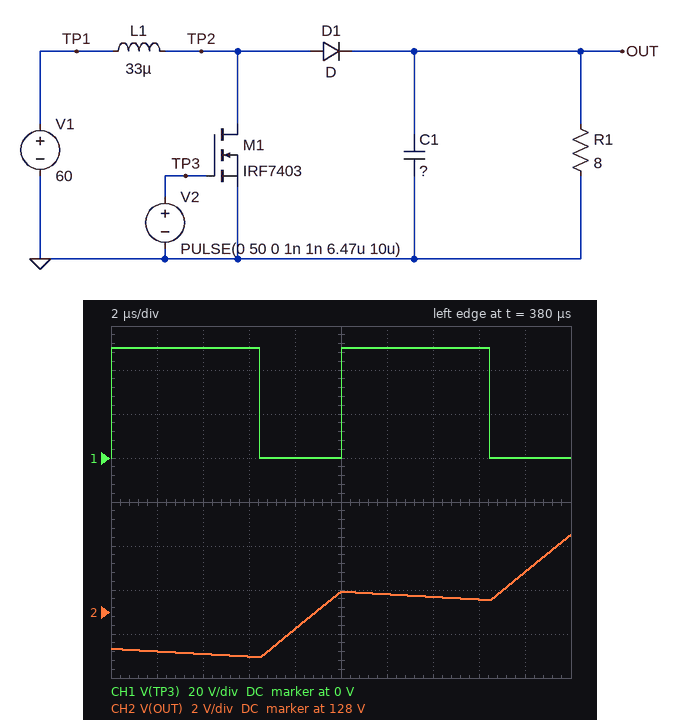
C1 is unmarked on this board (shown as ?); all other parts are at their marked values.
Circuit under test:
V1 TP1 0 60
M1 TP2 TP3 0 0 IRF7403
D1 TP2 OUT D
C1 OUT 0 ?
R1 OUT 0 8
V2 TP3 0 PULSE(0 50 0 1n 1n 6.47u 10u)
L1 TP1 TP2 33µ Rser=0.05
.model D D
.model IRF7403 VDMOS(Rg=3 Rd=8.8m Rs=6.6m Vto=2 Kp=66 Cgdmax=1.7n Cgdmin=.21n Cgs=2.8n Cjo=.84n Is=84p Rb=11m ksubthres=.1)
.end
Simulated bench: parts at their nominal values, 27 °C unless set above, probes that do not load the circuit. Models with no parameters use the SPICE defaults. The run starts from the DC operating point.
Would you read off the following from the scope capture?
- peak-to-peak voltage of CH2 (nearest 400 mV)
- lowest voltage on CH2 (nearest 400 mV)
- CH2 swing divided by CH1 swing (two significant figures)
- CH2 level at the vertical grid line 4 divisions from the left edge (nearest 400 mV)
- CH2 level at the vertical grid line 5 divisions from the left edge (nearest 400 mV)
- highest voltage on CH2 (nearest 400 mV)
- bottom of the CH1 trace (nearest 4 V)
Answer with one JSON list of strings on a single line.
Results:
["5.6 V", "126.0 V", "0.11", "127.2 V", "128.8 V", "131.6 V", "0 V"]
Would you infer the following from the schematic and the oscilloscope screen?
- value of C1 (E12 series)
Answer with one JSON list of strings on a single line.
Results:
["270 µF"]
